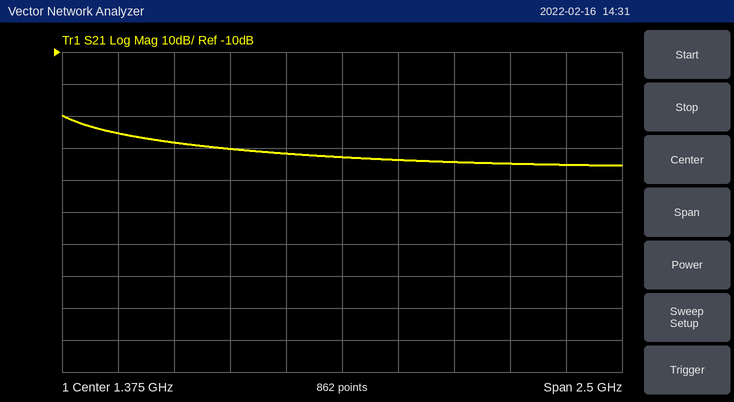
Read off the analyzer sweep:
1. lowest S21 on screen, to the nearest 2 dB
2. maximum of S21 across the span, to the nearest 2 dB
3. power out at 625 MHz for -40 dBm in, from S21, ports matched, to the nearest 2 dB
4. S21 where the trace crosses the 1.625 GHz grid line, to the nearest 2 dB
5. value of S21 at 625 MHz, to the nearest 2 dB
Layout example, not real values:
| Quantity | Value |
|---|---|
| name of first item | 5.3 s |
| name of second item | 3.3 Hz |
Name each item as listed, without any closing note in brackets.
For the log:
| Quantity | Value |
|---|---|
| lowest S21 on screen, to the nearest 2 dB | -46 dB |
| maximum of S21 across the span, to the nearest 2 dB | -30 dB |
| power out at 625 MHz for -40 dBm in, from S21, ports matched, to the nearest 2 dB | -78 dBm |
| S21 where the trace crosses the 1.625 GHz grid line, to the nearest 2 dB | -44 dB |
| value of S21 at 625 MHz, to the nearest 2 dB | -38 dB |
